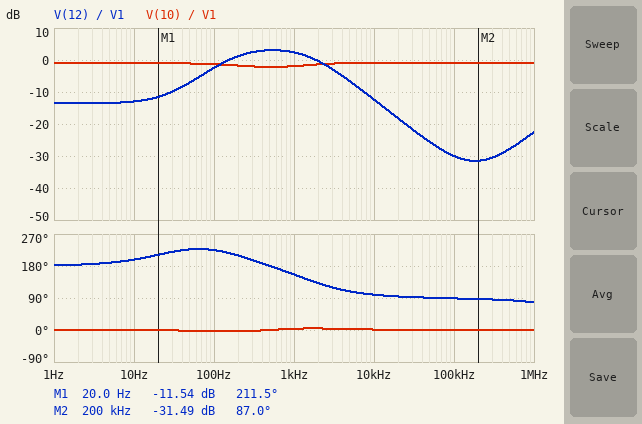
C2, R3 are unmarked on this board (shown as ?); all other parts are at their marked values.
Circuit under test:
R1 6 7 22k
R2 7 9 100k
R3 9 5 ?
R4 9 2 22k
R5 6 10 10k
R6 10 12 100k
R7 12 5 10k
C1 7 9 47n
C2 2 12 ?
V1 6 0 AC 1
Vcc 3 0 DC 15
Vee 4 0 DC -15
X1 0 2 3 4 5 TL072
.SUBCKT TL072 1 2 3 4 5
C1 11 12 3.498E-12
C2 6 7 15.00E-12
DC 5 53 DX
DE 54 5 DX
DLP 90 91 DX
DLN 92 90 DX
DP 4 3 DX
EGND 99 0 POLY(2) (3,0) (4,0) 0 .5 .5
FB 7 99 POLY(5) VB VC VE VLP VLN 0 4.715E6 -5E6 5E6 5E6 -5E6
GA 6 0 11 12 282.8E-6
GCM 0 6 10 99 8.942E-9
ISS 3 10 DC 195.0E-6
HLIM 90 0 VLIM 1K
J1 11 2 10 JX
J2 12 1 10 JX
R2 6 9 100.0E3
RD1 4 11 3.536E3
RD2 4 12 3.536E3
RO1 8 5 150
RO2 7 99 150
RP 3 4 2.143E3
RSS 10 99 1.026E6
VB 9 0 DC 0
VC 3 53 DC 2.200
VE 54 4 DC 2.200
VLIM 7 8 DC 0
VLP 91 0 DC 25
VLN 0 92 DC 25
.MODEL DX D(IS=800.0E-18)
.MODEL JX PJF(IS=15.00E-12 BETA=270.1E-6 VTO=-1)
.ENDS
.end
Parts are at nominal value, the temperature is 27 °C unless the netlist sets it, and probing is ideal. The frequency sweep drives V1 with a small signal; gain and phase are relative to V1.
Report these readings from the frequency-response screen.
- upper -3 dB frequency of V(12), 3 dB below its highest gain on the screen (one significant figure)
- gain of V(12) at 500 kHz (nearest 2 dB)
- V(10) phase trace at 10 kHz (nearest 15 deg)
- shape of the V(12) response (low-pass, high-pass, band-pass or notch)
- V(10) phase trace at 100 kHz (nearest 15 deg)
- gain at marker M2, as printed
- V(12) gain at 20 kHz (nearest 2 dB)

2 kHz
-28 dB
0 deg
band-pass
0 deg
-31.49 dB
-18 dB
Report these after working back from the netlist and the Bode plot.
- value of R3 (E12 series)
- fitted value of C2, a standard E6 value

39 kΩ
1 nF
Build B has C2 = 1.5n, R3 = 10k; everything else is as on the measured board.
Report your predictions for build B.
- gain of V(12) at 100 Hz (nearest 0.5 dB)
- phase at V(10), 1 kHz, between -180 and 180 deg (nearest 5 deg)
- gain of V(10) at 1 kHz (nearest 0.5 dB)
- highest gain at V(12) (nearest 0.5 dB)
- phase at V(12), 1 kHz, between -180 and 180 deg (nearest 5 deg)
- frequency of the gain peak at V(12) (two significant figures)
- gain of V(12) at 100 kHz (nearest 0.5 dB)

-16.0 dB
0 deg
-1.0 dB
-10.0 dB
165 deg
650 Hz
-38.0 dB
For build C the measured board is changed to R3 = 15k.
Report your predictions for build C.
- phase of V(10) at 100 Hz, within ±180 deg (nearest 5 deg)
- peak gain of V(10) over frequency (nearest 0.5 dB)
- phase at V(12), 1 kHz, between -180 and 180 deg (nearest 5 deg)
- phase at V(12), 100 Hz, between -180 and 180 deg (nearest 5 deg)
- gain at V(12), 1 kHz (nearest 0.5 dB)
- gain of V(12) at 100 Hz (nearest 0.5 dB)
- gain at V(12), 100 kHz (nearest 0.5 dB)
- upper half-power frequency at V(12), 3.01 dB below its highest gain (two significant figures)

0 deg
-0.5 dB
170 deg
-125 deg
-6.0 dB
-12.0 dB
-33.5 dB
3.1 kHz
